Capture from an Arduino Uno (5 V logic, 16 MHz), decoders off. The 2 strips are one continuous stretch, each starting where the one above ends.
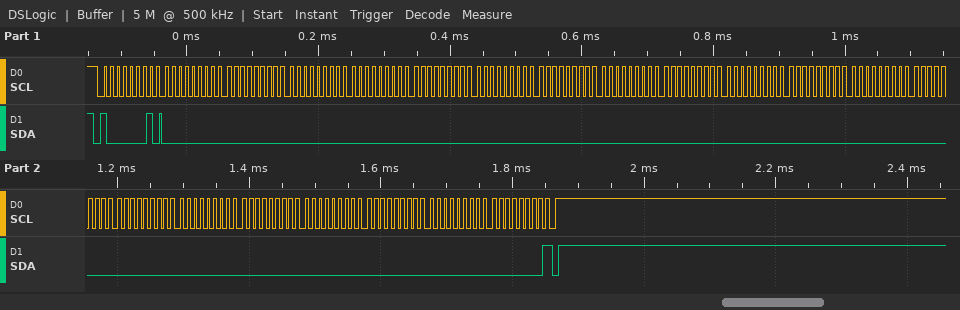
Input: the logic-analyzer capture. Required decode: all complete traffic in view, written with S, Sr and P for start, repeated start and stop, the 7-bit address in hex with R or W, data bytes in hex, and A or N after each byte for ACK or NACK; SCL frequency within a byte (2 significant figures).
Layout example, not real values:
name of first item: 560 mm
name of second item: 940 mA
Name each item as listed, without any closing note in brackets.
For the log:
all complete traffic in view, written with S, Sr and P for start, repeated start and stop, the 7-bit address in hex with R or W, data bytes in hex, and A or N after each byte for ACK or NACK: S 40R A 00 A 00 A 00 A 00 A 00 A 00 A 00 A 00 A 00 A 00 A 00 A 00 A 00 A 00 A 00 A 00 A 00 A 00 A 00 A 00 N P
SCL frequency within a byte: 100 kHz
